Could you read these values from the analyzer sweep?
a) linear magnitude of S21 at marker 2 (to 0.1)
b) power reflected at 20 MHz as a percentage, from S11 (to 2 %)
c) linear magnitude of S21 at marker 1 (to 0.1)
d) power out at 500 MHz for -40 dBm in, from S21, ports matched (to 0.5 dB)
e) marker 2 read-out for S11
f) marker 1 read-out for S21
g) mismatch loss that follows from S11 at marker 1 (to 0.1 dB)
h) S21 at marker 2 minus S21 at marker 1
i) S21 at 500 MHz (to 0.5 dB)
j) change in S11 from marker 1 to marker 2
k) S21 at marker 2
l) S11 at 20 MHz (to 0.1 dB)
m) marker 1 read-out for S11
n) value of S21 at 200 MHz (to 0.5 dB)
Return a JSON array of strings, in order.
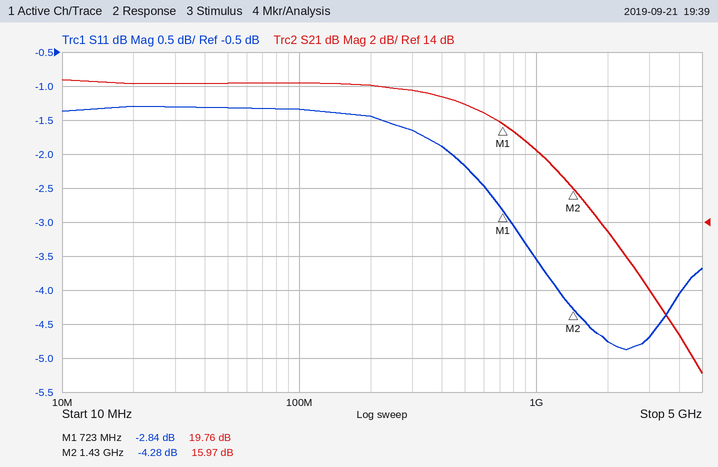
["6.3", "74 %", "9.7", "-19.0 dBm", "-4.28 dB", "19.76 dB", "3.2 dB", "-3.79 dB", "21.0 dB", "-1.44 dB", "15.97 dB", "-1.3 dB", "-2.84 dB", "22.0 dB"]
